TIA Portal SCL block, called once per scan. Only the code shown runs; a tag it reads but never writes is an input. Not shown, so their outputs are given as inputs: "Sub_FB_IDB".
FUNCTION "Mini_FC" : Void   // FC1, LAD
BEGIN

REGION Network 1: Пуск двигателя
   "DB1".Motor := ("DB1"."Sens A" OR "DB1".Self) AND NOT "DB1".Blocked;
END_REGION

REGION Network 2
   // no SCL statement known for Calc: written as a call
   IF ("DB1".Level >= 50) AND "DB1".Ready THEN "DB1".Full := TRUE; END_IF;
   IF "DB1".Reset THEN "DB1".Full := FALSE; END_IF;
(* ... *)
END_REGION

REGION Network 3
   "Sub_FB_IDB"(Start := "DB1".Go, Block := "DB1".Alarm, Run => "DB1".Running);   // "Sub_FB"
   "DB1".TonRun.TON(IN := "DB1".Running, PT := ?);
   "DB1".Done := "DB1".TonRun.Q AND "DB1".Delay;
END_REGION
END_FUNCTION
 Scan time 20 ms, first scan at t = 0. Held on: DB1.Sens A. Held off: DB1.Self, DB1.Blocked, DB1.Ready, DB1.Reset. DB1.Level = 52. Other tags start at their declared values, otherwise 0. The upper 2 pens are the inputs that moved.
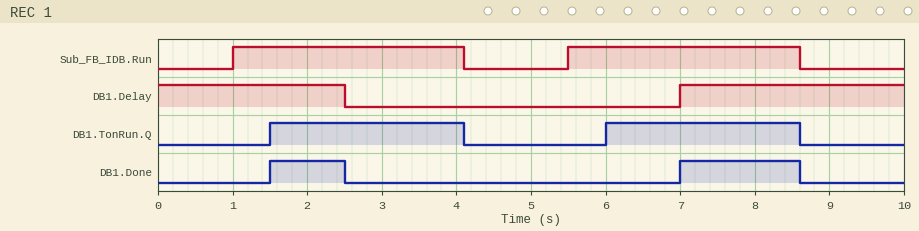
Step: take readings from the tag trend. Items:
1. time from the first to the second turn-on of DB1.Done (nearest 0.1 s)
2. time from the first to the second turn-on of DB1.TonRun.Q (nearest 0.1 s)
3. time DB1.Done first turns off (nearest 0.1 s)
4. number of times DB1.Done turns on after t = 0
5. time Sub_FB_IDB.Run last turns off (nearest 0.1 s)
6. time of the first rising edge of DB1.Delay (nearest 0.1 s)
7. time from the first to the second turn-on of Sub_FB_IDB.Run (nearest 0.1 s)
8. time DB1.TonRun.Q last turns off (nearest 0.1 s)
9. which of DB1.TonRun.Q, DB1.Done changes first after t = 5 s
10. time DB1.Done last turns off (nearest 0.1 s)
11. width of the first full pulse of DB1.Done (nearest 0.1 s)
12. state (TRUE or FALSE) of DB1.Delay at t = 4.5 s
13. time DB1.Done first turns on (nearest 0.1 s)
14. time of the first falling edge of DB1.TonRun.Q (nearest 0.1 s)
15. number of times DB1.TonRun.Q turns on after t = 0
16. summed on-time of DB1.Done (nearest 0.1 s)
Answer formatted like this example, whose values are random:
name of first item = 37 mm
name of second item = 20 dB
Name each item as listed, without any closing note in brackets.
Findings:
time from the first to the second turn-on of DB1.Done = 5.5 s
time from the first to the second turn-on of DB1.TonRun.Q = 4.5 s
time DB1.Done first turns off = 2.5 s
number of times DB1.Done turns on after t = 0 = 2
time Sub_FB_IDB.Run last turns off = 8.6 s
time of the first rising edge of DB1.Delay = 7.0 s
time from the first to the second turn-on of Sub_FB_IDB.Run = 4.5 s
time DB1.TonRun.Q last turns off = 8.6 s
which of DB1.TonRun.Q, DB1.Done changes first after t = 5 s = DB1.TonRun.Q
time DB1.Done last turns off = 8.6 s
width of the first full pulse of DB1.Done = 1.0 s
state (TRUE or FALSE) of DB1.Delay at t = 4.5 s = FALSE
time DB1.Done first turns on = 1.5 s
time of the first falling edge of DB1.TonRun.Q = 4.1 s
number of times DB1.TonRun.Q turns on after t = 0 = 2
summed on-time of DB1.Done = 2.6 s
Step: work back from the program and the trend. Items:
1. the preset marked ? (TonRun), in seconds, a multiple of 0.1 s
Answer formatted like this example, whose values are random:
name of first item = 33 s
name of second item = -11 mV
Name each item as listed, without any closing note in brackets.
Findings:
the preset marked ? (TonRun), in seconds, a multiple of 0.1 s = 0.5 s
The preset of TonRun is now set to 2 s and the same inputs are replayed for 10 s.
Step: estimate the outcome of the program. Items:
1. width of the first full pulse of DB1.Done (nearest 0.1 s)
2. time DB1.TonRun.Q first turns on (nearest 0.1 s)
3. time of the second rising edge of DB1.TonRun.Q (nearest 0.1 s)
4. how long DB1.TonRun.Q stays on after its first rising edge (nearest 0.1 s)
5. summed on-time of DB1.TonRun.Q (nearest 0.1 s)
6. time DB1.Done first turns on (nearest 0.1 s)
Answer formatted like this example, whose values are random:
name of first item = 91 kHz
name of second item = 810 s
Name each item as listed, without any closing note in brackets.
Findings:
width of the first full pulse of DB1.Done = 1.1 s
time DB1.TonRun.Q first turns on = 3.0 s
time of the second rising edge of DB1.TonRun.Q = 7.5 s
how long DB1.TonRun.Q stays on after its first rising edge = 1.1 s
summed on-time of DB1.TonRun.Q = 2.2 s
time DB1.Done first turns on = 7.5 s
